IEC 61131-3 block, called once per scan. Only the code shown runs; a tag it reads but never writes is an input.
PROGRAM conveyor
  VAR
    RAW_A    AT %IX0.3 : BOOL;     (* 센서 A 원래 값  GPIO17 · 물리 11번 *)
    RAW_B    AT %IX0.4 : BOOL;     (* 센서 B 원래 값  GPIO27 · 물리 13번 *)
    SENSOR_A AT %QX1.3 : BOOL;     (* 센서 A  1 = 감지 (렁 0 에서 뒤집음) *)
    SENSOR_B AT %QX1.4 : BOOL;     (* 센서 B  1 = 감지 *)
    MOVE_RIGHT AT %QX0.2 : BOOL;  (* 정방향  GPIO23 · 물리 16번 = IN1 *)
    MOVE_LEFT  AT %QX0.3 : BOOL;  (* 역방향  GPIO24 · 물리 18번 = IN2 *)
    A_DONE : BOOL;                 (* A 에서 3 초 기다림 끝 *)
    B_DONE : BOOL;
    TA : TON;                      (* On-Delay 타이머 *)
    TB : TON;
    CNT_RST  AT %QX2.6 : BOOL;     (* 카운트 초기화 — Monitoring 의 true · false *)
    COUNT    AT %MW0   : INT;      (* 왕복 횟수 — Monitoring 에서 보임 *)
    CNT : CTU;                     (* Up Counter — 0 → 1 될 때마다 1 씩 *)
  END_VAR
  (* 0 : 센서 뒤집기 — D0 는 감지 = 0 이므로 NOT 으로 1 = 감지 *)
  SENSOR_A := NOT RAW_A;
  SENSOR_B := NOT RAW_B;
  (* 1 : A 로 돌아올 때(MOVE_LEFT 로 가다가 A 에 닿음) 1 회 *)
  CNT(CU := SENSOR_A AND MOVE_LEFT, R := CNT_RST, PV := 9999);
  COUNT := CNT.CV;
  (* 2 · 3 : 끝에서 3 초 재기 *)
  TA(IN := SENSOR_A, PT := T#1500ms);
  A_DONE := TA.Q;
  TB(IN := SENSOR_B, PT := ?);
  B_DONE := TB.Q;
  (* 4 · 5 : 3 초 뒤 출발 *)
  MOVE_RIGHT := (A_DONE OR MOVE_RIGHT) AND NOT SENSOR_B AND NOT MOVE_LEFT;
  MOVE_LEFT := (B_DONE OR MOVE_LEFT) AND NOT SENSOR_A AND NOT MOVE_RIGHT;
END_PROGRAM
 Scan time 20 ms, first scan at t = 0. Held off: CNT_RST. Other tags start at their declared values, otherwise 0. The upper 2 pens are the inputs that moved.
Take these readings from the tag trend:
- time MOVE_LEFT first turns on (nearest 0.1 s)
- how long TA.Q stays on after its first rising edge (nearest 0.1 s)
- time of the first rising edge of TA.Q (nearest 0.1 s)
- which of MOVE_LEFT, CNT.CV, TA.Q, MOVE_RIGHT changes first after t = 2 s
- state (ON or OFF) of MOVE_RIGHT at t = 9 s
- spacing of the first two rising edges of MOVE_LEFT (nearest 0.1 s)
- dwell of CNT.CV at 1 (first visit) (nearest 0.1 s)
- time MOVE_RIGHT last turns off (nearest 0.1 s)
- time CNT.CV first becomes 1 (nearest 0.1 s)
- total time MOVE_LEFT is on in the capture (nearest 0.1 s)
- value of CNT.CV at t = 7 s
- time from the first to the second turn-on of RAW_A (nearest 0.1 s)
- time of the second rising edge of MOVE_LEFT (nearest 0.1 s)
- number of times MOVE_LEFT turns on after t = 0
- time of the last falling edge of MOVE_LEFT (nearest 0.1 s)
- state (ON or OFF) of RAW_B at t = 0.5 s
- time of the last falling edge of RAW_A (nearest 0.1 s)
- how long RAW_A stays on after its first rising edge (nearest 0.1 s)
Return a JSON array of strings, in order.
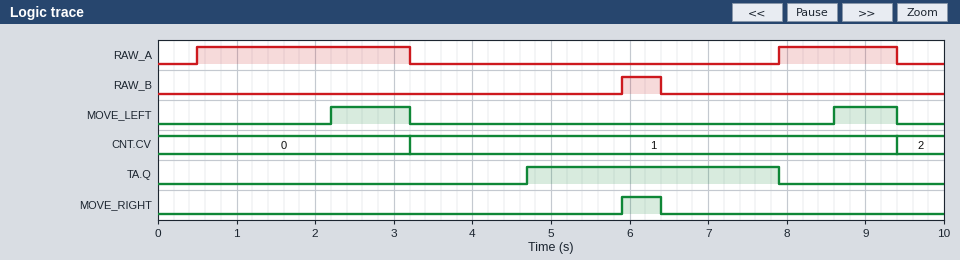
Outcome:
["2.2 s", "3.2 s", "4.7 s", "MOVE_LEFT", "OFF", "6.4 s", "6.2 s", "6.4 s", "3.2 s", "1.8 s", "1", "7.4 s", "8.6 s", "2", "9.4 s", "OFF", "9.4 s", "2.7 s"]
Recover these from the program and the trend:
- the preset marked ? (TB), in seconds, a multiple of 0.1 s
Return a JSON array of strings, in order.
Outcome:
["2.2 s"]
